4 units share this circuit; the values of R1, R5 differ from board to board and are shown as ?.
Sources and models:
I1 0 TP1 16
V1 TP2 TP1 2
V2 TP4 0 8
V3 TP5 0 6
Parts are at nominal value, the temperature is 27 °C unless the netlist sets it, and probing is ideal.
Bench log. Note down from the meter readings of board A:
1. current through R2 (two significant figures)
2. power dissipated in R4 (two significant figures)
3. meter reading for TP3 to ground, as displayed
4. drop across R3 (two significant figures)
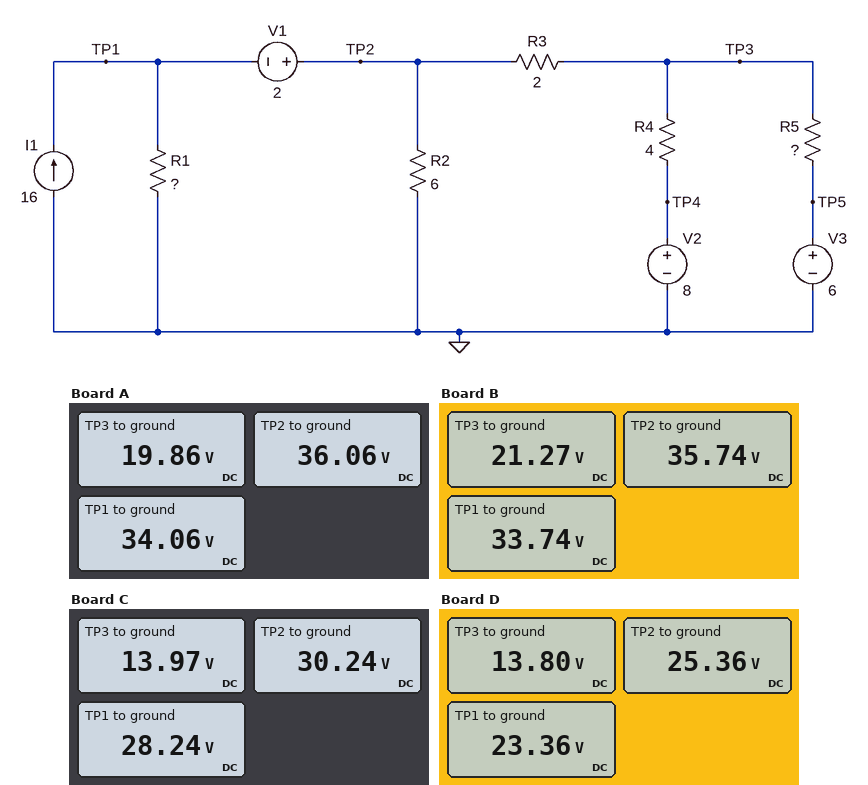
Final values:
6.0 A
35 W
19.86 V
16 V
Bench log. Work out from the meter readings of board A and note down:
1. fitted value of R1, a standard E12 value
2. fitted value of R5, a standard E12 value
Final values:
18 Ω
2.7 Ω
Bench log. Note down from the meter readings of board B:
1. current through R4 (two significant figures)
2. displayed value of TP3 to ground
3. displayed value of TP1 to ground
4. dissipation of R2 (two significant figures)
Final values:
3.3 A
21.27 V
33.74 V
210 W
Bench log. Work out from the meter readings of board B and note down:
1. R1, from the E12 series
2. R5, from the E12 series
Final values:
12 Ω
3.9 Ω
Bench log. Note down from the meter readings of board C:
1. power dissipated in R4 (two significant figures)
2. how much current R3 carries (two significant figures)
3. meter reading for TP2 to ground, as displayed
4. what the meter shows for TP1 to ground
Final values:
8.9 W
8.1 A
30.24 V
28.24 V
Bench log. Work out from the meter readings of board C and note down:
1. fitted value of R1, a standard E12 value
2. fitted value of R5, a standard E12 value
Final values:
10 Ω
1.2 Ω
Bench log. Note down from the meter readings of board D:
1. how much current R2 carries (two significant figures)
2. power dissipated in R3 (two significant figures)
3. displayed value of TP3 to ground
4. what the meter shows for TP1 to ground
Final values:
4.2 A
67 W
13.80 V
23.36 V
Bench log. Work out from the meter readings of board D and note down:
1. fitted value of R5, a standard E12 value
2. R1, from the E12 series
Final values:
1.8 Ω
3.9 Ω
